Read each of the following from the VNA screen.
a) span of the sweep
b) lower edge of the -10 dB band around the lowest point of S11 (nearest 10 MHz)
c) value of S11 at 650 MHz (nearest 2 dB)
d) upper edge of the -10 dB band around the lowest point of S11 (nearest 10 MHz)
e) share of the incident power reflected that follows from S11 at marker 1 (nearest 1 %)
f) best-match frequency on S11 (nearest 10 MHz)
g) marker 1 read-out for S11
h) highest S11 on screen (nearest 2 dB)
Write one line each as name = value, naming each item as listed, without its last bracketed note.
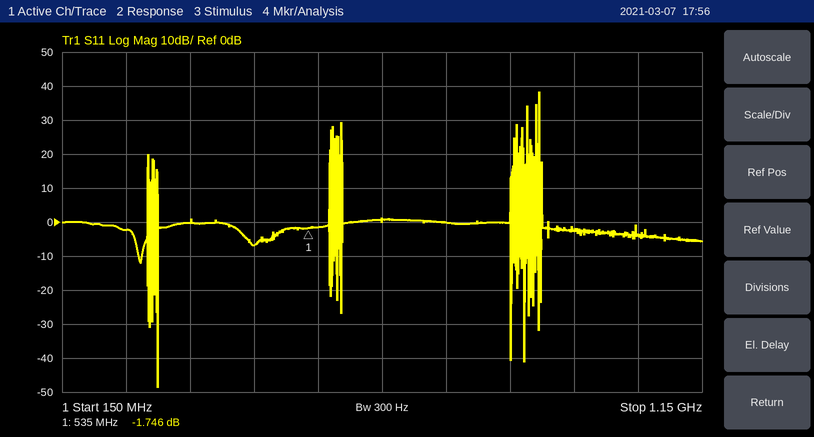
span of the sweep = 1 GHz
lower edge of the -10 dB band around the lowest point of S11 = 300 MHz
value of S11 at 650 MHz = 0 dB
upper edge of the -10 dB band around the lowest point of S11 = 300 MHz
share of the incident power reflected that follows from S11 at marker 1 = 67 %
best-match frequency on S11 = 300 MHz
marker 1 read-out for S11 = -1.746 dB
highest S11 on screen = 38 dB
